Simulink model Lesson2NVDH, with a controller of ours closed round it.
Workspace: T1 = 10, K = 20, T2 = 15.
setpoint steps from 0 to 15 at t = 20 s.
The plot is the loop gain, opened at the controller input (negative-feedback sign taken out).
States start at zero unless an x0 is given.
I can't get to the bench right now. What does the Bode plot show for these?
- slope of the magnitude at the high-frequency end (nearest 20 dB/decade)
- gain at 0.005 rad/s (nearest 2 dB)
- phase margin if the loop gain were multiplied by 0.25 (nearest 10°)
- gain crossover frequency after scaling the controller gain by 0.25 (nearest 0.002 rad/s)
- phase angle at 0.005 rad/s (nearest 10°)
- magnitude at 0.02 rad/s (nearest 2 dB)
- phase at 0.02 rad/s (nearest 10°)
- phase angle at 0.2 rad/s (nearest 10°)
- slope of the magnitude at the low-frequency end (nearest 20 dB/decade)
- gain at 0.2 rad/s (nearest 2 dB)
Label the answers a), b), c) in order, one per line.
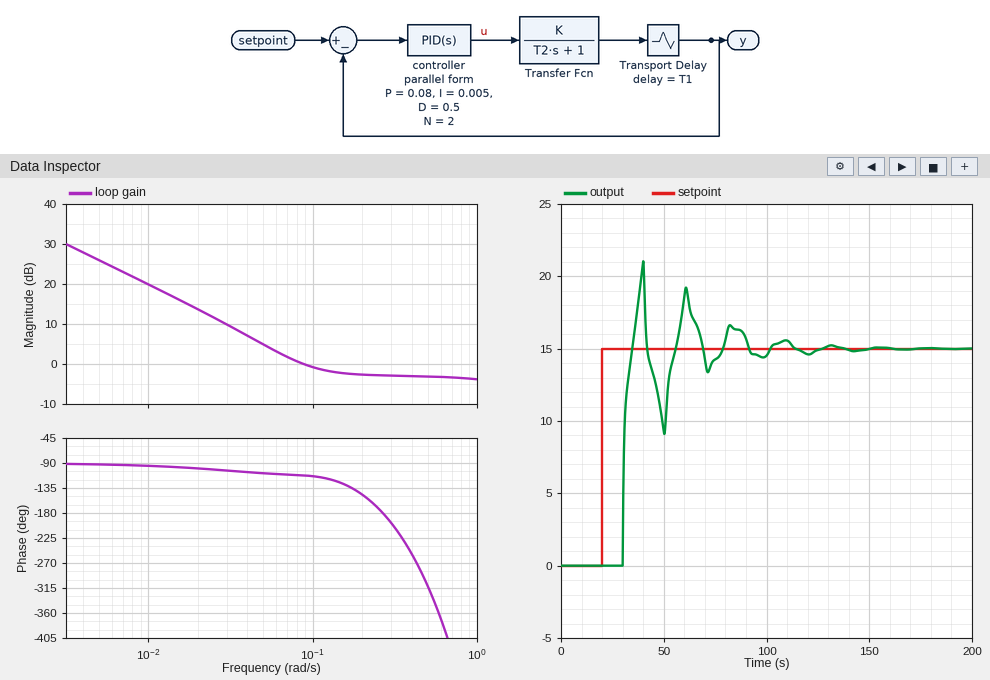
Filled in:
a) 0 dB/decade
b) 26 dB
c) 80°
d) 0.024 rad/s
e) -90°
f) 14 dB
g) -100°
h) -150°
i) -20 dB/decade
j) -2 dB
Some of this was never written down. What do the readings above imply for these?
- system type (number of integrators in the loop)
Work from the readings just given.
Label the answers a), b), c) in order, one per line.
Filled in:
a) 1
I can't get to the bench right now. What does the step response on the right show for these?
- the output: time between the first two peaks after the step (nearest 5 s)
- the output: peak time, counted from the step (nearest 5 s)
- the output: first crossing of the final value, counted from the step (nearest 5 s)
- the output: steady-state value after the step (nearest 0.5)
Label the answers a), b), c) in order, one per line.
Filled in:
a) 20 s
b) 20 s
c) 15 s
d) 15.0
